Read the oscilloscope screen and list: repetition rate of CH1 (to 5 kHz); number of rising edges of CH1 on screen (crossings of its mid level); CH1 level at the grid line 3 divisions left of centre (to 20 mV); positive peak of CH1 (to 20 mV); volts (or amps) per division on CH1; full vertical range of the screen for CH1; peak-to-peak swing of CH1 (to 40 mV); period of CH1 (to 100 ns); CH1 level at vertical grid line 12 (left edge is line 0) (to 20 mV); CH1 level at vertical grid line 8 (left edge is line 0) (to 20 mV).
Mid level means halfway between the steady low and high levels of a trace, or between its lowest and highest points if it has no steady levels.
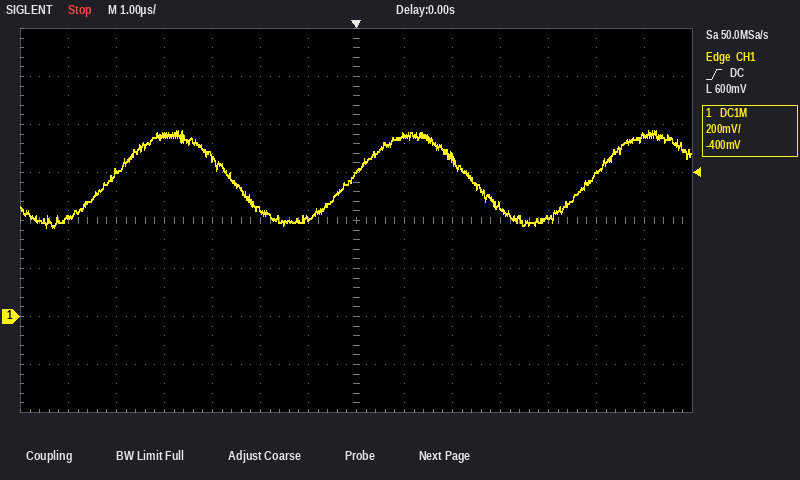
200 kHz
3
660 mV
780 mV
200 mV
1.6 V
400 mV
5.0 µs
600 mV
760 mV
